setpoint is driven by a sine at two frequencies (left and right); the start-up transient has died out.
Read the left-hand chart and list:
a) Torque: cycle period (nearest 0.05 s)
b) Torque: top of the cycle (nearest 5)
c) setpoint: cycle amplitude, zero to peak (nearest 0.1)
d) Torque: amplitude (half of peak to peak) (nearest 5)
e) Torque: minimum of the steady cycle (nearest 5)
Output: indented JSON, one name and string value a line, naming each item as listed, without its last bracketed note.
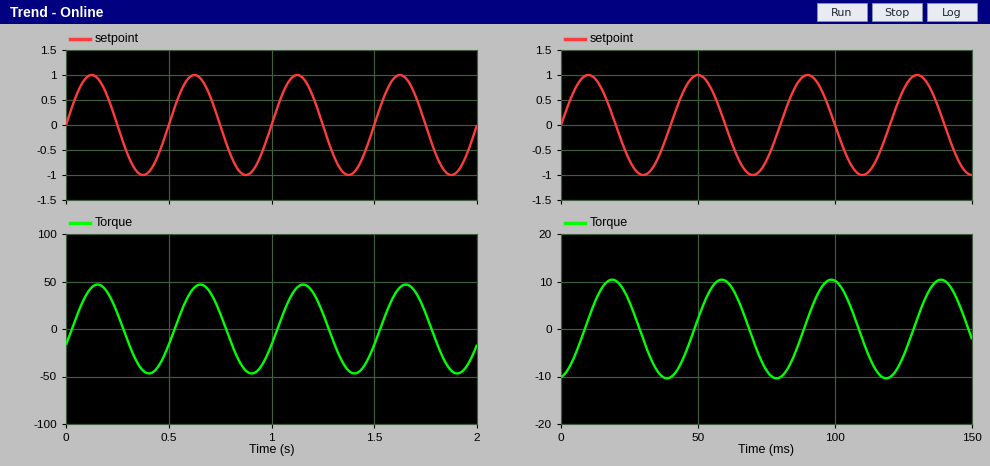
{
  "Torque: cycle period": "0.50 s",
  "Torque: top of the cycle": "45",
  "setpoint: cycle amplitude, zero to peak": "1.0",
  "Torque: amplitude (half of peak to peak)": "45",
  "Torque: minimum of the steady cycle": "-45"
}
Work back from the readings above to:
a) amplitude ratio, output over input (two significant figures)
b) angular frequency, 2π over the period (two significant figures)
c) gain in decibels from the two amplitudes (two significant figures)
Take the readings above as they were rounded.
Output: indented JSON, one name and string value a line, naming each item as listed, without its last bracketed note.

{
  "amplitude ratio, output over input": "45",
  "angular frequency, 2π over the period": "13 rad/s",
  "gain in decibels from the two amplitudes": "33 dB"
}
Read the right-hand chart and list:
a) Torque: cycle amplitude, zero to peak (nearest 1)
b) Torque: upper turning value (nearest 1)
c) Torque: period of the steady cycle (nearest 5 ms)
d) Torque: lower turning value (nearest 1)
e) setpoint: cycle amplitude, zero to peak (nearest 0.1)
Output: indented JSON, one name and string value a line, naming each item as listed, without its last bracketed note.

{
  "Torque: cycle amplitude, zero to peak": "10",
  "Torque: upper turning value": "10",
  "Torque: period of the steady cycle": "40 ms",
  "Torque: lower turning value": "-10",
  "setpoint: cycle amplitude, zero to peak": "1.0"
}
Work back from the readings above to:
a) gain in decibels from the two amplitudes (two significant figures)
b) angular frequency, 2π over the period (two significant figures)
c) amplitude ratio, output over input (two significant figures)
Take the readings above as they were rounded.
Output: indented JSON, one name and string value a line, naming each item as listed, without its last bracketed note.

{
  "gain in decibels from the two amplitudes": "20 dB",
  "angular frequency, 2π over the period": "0.16 rad/ms",
  "amplitude ratio, output over input": "10"
}
